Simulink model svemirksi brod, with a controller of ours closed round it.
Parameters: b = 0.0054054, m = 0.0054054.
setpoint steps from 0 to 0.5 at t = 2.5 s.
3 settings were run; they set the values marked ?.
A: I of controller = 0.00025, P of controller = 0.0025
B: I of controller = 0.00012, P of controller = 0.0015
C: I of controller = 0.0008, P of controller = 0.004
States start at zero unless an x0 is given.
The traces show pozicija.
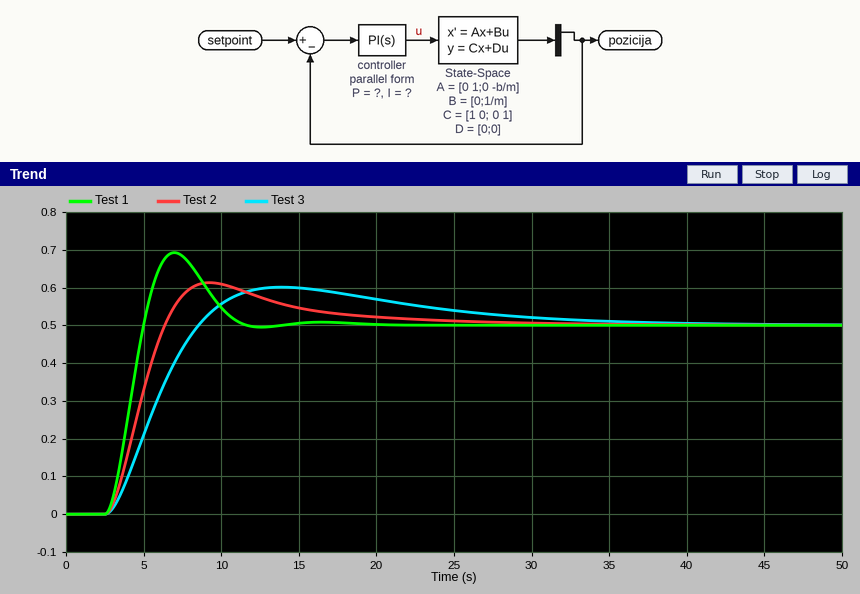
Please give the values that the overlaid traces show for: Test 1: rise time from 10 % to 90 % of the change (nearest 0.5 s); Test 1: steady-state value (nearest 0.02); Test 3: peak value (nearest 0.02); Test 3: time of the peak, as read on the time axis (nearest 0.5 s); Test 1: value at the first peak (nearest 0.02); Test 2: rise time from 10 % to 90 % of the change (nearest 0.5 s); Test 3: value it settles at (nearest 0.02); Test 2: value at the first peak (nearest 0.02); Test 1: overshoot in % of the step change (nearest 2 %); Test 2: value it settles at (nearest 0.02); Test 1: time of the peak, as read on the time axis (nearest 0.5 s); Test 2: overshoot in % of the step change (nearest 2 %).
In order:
1.5 s
0.50
0.60
14.0 s
0.70
2.5 s
0.50
0.62
38 %
0.50
7.0 s
22 %
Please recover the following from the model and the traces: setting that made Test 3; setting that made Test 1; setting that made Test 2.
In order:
B
C
A
